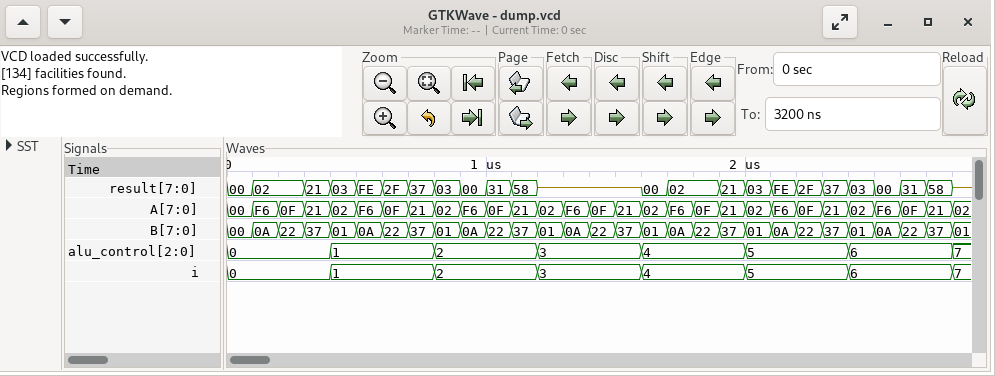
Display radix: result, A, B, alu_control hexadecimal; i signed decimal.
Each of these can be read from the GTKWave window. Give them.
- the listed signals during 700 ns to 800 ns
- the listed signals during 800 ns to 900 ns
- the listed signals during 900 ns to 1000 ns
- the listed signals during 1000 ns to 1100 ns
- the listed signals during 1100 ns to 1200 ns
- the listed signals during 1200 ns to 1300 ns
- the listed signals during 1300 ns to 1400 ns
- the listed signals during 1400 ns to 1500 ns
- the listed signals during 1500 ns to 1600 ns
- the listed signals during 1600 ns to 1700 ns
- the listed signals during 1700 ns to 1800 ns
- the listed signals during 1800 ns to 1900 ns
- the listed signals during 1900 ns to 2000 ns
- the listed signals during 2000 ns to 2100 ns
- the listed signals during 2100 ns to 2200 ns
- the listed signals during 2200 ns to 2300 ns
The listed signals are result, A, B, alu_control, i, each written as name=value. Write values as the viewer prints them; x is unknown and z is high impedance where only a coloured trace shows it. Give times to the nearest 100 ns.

result=37, A=21, B=37, alu_control=1, i=1
result=03, A=02, B=01, alu_control=2, i=2
result=00, A=F6, B=0A, alu_control=2, i=2
result=31, A=0F, B=22, alu_control=2, i=2
result=58, A=21, B=37, alu_control=2, i=2
result=z, A=02, B=01, alu_control=3, i=3
result=z, A=F6, B=0A, alu_control=3, i=3
result=z, A=0F, B=22, alu_control=3, i=3
result=z, A=21, B=37, alu_control=3, i=3
result=00, A=02, B=01, alu_control=4, i=4
result=02, A=F6, B=0A, alu_control=4, i=4
result=02, A=0F, B=22, alu_control=4, i=4
result=21, A=21, B=37, alu_control=4, i=4
result=03, A=02, B=01, alu_control=5, i=5
result=FE, A=F6, B=0A, alu_control=5, i=5
result=2F, A=0F, B=22, alu_control=5, i=5
